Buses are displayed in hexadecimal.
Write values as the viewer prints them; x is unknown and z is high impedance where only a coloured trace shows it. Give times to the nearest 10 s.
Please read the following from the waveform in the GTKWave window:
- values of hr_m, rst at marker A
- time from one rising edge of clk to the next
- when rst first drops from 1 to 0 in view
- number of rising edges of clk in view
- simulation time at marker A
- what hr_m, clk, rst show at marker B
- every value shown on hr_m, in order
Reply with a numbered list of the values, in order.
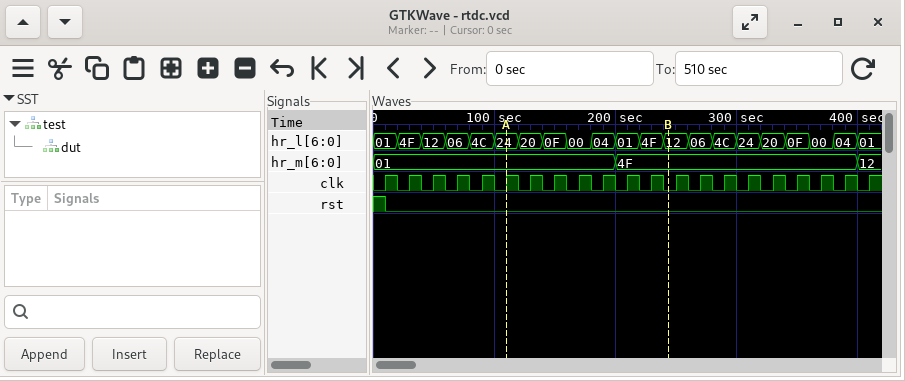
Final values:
1. hr_m=01, rst=0
2. 20 s
3. 10 s
4. 21
5. 110 s
6. hr_m=4F, clk=0, rst=0
7. 01, 4F, 12
